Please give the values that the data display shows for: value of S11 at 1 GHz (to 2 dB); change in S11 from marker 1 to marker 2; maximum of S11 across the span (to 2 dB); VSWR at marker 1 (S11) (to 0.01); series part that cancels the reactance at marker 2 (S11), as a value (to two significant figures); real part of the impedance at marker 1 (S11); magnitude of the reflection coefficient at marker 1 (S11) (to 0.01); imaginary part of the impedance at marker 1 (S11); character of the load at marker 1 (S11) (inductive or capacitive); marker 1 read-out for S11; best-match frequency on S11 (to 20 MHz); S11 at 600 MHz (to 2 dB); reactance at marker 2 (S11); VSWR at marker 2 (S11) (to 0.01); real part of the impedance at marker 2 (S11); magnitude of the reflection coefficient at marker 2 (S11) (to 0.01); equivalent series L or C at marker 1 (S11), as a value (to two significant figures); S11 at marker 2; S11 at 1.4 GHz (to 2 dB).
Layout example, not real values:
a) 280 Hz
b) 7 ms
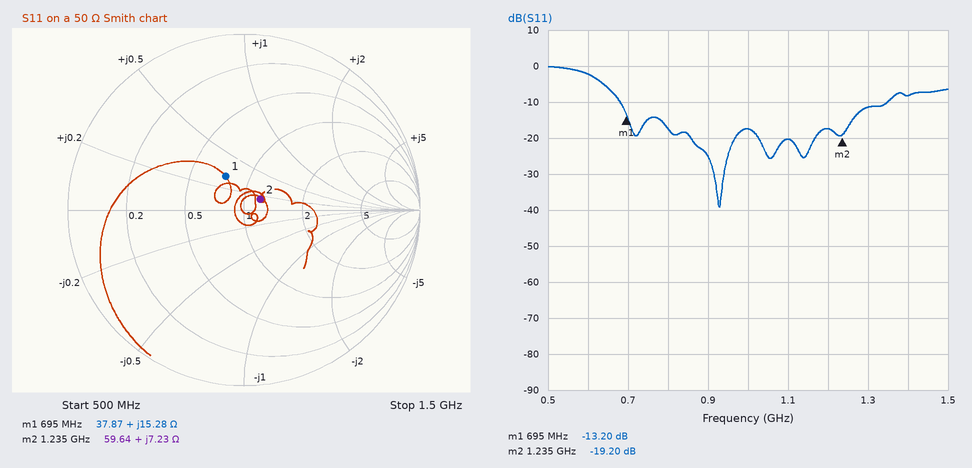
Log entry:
a) -18 dB
b) -6.00 dB
c) 0 dB
d) 1.56
e) 18 pF
f) 37.87 Ω
g) 0.22
h) +15.28 Ω
i) inductive
j) -13.20 dB
k) 920 MHz
l) -2 dB
m) +7.23 Ω
n) 1.25
o) 59.64 Ω
p) 0.11
q) 3.5 nH
r) -19.20 dB
s) -8 dB
